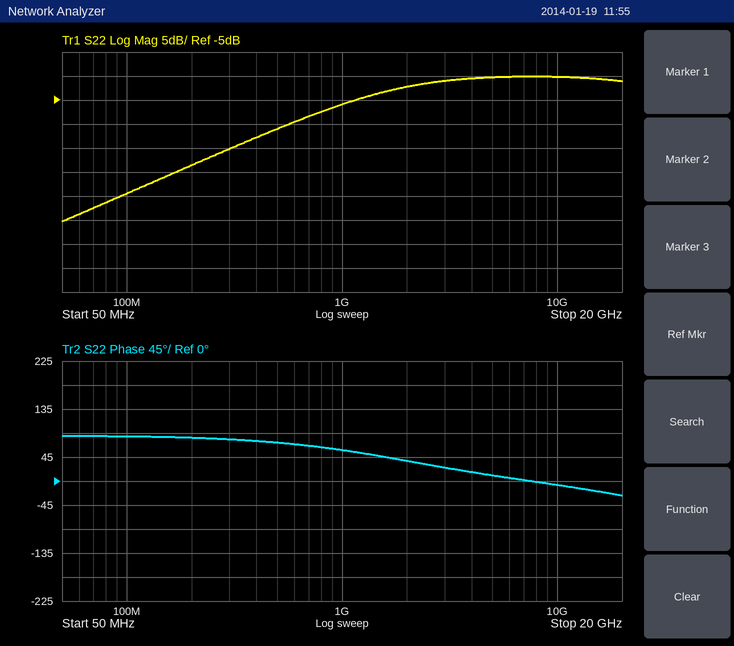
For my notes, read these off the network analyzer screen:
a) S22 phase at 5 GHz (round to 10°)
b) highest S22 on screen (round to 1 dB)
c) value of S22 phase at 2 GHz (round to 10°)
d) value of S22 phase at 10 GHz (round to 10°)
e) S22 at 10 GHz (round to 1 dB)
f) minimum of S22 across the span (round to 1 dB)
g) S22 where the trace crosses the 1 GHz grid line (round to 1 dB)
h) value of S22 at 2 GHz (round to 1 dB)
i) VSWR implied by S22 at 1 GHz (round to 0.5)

10°
0 dB
40°
-10°
0 dB
-30 dB
-6 dB
-2 dB
3.0
